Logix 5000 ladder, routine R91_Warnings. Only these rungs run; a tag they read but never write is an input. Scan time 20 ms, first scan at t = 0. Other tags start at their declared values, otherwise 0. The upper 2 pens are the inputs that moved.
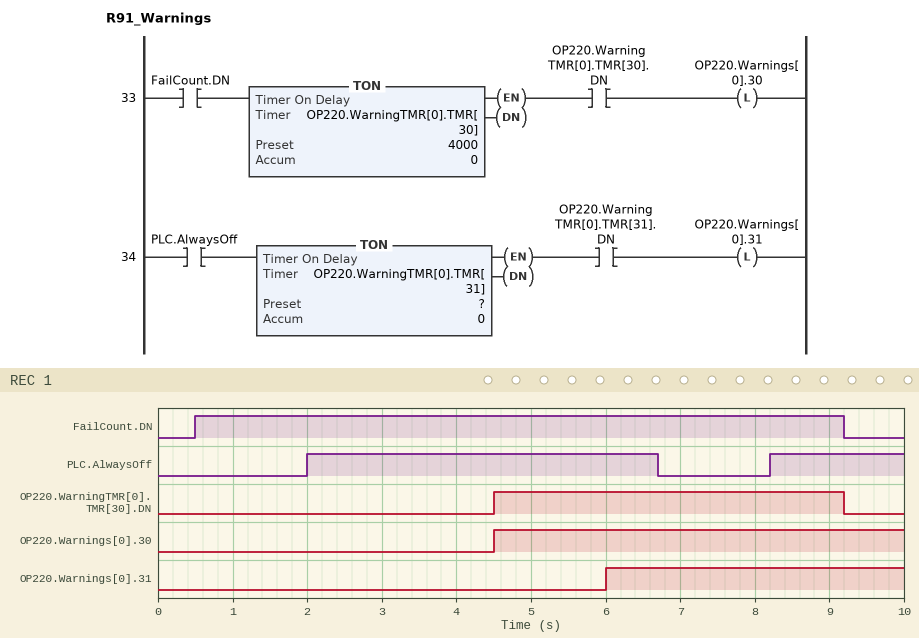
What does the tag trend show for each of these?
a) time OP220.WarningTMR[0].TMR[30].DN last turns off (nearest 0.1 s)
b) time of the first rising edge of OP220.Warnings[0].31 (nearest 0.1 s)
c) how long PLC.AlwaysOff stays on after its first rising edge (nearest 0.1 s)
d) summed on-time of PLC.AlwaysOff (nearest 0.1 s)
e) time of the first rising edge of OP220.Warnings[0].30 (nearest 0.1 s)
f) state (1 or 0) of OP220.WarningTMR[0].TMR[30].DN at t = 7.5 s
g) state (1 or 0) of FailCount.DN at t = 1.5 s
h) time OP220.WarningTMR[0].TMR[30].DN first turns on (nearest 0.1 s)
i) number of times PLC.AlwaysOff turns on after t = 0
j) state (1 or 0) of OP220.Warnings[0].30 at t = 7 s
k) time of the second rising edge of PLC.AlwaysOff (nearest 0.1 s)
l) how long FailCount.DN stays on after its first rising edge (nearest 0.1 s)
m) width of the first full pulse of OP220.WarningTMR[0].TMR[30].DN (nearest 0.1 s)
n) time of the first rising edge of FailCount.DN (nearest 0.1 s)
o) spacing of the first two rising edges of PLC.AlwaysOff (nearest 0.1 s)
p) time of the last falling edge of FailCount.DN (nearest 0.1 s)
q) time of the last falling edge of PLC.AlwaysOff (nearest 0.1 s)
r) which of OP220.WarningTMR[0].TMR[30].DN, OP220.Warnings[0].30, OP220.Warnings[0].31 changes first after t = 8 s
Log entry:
9.2 s
6.0 s
4.7 s
6.5 s
4.5 s
1
1
4.5 s
2
1
8.2 s
8.7 s
4.7 s
0.5 s
6.2 s
9.2 s
6.7 s
OP220.WarningTMR[0].TMR[30].DN
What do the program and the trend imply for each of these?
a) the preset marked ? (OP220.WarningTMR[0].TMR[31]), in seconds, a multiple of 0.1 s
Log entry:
4.0 s
